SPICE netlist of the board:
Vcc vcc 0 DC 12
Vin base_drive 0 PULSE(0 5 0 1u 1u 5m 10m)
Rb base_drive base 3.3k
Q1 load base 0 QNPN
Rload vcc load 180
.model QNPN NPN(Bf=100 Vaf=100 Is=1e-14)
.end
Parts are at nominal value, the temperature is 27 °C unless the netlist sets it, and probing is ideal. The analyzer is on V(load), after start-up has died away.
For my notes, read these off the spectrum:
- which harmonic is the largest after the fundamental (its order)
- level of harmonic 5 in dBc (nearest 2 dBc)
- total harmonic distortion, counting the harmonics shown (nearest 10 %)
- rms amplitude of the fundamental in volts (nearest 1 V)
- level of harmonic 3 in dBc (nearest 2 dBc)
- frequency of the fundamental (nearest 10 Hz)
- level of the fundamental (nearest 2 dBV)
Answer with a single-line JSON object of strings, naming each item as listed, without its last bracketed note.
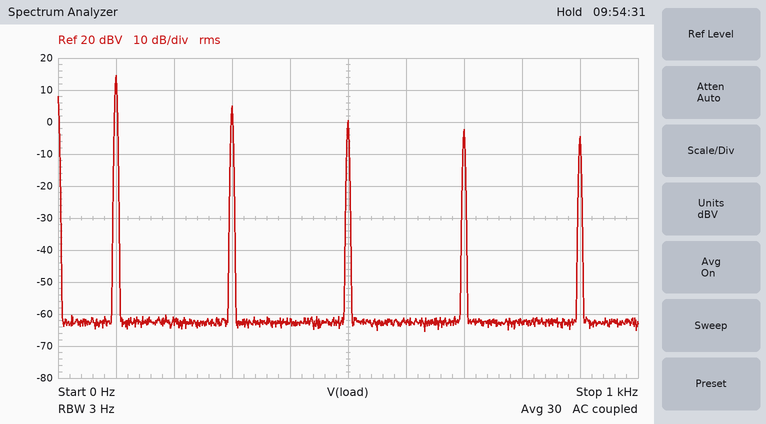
{"which harmonic is the largest after the fundamental": "3", "level of harmonic 5 in dBc": "-14 dBc", "total harmonic distortion, counting the harmonics shown": "40 %", "rms amplitude of the fundamental in volts": "5 V", "level of harmonic 3 in dBc": "-10 dBc", "frequency of the fundamental": "100 Hz", "level of the fundamental": "14 dBV"}
